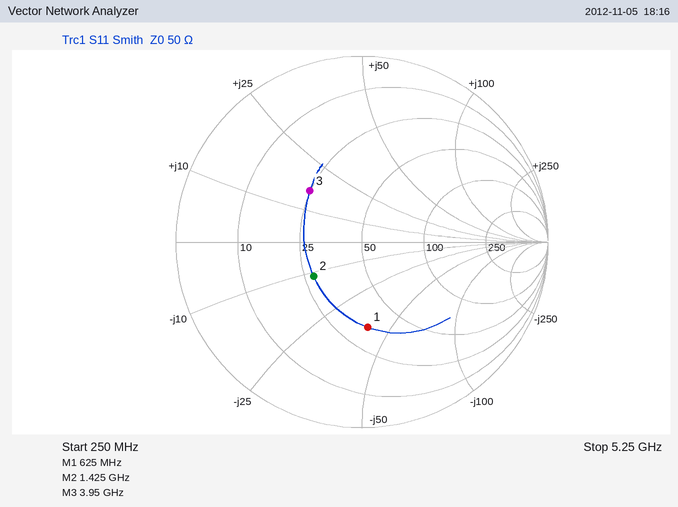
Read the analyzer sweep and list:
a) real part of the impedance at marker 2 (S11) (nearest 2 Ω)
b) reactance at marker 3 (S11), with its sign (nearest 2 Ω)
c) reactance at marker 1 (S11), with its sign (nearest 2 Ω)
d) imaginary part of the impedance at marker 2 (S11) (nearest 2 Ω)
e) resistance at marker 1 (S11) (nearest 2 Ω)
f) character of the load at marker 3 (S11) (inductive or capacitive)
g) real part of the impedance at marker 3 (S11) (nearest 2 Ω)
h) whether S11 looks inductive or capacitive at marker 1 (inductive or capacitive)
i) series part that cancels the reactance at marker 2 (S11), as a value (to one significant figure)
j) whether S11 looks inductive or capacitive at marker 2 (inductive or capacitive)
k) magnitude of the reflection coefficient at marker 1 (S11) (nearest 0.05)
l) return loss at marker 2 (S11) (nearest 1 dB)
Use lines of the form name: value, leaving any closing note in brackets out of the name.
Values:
real part of the impedance at marker 2 (S11): 28 Ω
reactance at marker 3 (S11), with its sign: +16 Ω
reactance at marker 1 (S11), with its sign: -40 Ω
imaginary part of the impedance at marker 2 (S11): -12 Ω
resistance at marker 1 (S11): 34 Ω
character of the load at marker 3 (S11): inductive
real part of the impedance at marker 3 (S11): 24 Ω
whether S11 looks inductive or capacitive at marker 1: capacitive
series part that cancels the reactance at marker 2 (S11), as a value: 1 nH
whether S11 looks inductive or capacitive at marker 2: capacitive
magnitude of the reflection coefficient at marker 1 (S11): 0.45
return loss at marker 2 (S11): 10 dB
